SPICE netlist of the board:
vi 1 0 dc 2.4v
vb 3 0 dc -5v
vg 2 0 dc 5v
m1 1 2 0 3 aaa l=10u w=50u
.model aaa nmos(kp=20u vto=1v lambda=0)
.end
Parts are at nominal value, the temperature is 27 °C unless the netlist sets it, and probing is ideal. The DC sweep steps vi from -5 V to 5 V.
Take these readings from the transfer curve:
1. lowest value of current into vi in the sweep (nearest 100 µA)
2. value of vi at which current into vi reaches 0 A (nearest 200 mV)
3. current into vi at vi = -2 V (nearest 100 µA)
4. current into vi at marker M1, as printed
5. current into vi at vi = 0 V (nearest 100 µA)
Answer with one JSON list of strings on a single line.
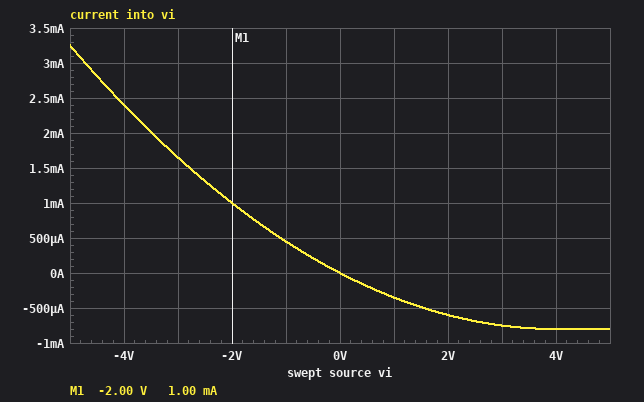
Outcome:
["-800 µA", "0 V", "1.0 mA", "1.00 mA", "0 A"]
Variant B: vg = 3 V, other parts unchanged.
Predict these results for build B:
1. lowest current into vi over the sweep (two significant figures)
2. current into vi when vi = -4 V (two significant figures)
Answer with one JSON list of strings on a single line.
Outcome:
["-200 µA", "1.6 mA"]
